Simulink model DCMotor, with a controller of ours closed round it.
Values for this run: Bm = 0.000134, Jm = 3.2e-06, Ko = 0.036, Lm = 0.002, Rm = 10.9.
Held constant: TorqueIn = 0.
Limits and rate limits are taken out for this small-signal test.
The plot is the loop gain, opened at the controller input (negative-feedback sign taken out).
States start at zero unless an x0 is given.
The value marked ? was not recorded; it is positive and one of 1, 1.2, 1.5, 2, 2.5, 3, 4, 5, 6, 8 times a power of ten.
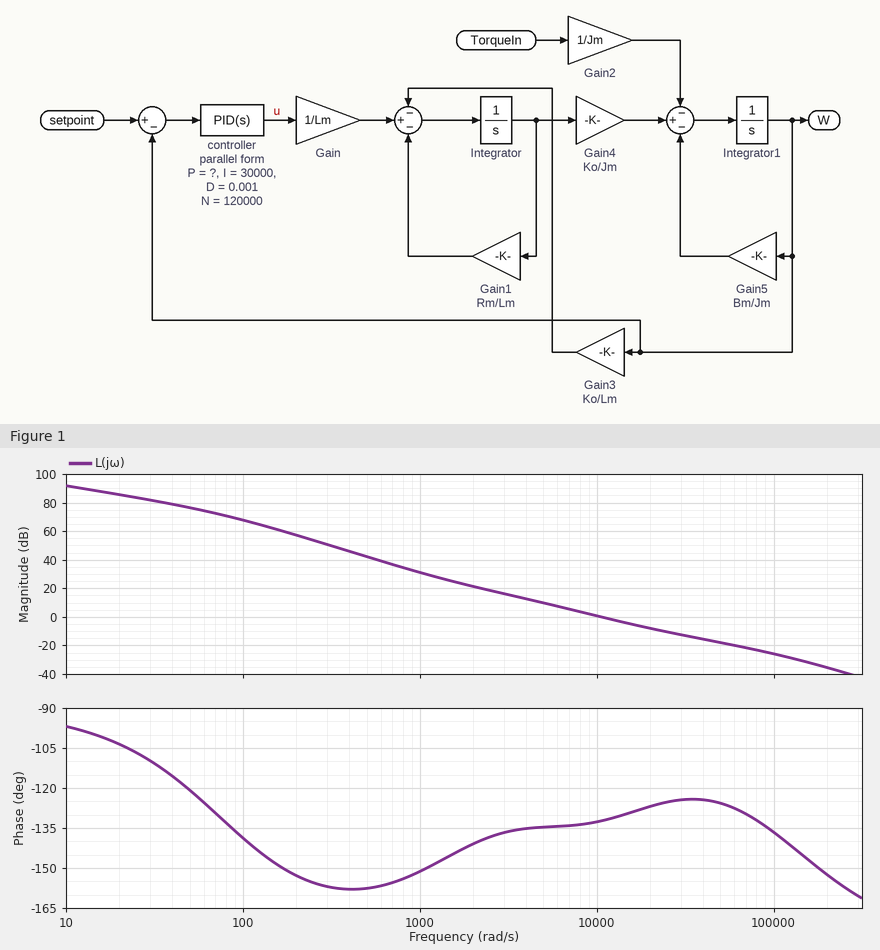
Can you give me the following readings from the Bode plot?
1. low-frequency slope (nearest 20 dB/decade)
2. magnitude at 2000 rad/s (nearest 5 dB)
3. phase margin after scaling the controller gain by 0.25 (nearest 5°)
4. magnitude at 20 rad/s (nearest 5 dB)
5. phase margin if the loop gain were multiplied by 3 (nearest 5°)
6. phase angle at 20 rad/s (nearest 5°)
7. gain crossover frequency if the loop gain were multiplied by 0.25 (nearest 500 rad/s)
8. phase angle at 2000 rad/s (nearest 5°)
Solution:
-20 dB/decade
20 dB
45°
85 dB
55°
-105°
4000 rad/s
-140°
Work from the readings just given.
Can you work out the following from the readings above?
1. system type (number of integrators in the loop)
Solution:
1
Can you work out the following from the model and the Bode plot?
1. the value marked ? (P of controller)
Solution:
20
